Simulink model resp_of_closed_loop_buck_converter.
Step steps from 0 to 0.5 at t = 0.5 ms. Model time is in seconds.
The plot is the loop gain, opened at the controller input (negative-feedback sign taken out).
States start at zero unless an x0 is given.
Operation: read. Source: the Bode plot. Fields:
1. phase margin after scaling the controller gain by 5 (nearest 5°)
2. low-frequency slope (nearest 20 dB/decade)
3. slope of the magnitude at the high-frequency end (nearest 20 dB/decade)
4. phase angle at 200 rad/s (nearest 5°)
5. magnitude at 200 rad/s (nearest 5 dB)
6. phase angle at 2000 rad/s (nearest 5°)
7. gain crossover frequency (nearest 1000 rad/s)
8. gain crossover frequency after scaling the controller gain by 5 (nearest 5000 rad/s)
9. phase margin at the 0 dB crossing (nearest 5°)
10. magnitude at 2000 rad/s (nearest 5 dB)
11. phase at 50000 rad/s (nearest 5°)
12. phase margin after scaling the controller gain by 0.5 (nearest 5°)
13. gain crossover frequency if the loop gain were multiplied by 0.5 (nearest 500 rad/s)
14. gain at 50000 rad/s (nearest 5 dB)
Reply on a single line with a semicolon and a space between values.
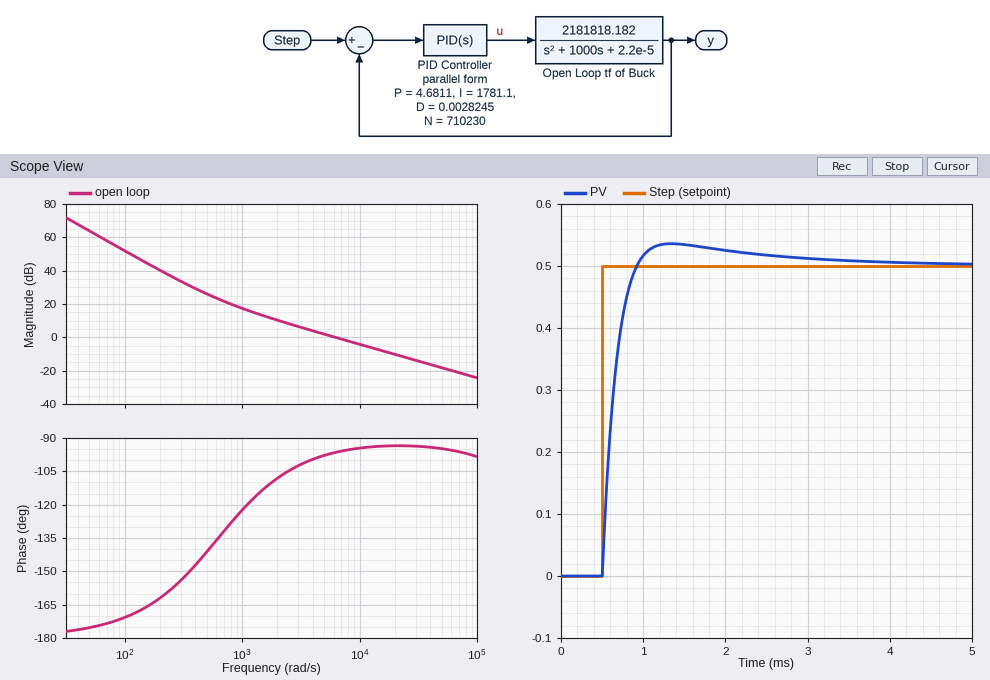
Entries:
85°; -40 dB/decade; -20 dB/decade; -160°; 40 dB; -110°; 6000 rad/s; 30000 rad/s; 85°; 10 dB; -95°; 80°; 3000 rad/s; -20 dB
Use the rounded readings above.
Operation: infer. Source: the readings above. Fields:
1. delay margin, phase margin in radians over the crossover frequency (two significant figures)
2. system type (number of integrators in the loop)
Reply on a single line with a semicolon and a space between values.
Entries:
0.00025 s; 2
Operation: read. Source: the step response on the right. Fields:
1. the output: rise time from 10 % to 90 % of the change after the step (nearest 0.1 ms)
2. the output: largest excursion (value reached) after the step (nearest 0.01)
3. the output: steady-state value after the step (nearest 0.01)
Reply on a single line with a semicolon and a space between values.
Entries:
0.3 ms; 0.54; 0.50
